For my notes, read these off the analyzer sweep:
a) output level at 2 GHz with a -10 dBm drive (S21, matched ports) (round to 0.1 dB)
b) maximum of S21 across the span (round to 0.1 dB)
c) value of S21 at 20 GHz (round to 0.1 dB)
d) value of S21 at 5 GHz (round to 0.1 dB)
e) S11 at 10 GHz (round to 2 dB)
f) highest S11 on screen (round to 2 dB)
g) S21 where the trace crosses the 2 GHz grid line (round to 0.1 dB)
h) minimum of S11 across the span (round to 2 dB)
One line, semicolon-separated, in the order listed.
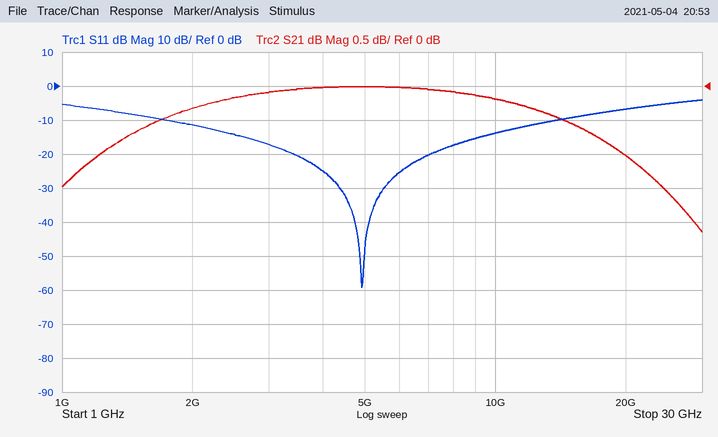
-10.3 dBm; 0.0 dB; -1.0 dB; 0.0 dB; -14 dB; -4 dB; -0.3 dB; -60 dB
